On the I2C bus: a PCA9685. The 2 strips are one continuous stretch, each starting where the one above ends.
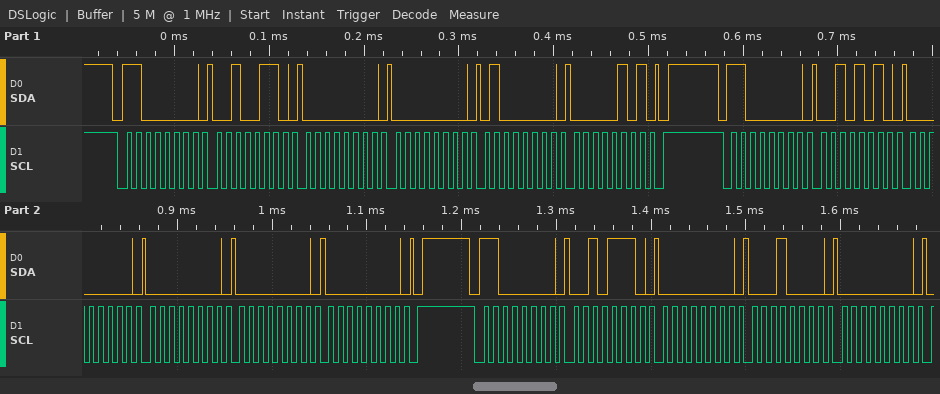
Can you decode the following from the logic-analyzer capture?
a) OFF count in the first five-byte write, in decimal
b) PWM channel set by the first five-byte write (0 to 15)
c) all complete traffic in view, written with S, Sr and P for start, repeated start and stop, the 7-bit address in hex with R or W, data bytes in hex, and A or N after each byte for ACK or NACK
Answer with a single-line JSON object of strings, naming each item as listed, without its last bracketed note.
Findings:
{"OFF count in the first five-byte write, in decimal": "1344", "PWM channel set by the first five-byte write": "8", "all complete traffic in view, written with S, Sr and P for start, repeated start and stop, the 7-bit address in hex with R or W, data bytes in hex, and A or N after each byte for ACK or NACK": "S 60W A 26 A 00 A 00 A 40 A 05 A P S 60W A 2A A 00 A 00 A 00 A 00 A P S 60W A 2E A 00 A 10 A 00 A"}
